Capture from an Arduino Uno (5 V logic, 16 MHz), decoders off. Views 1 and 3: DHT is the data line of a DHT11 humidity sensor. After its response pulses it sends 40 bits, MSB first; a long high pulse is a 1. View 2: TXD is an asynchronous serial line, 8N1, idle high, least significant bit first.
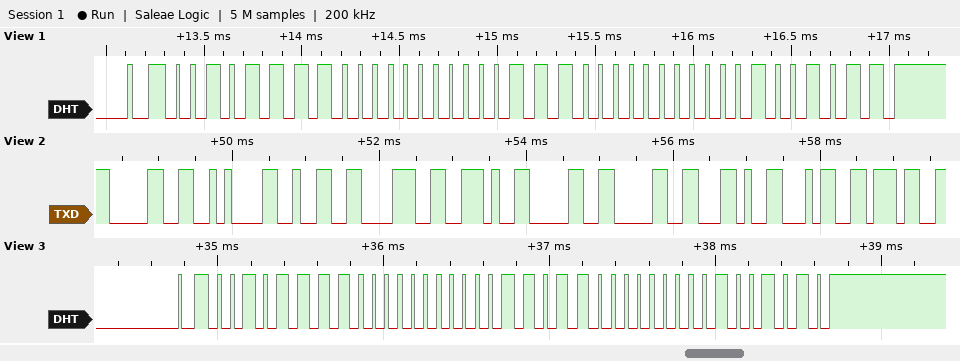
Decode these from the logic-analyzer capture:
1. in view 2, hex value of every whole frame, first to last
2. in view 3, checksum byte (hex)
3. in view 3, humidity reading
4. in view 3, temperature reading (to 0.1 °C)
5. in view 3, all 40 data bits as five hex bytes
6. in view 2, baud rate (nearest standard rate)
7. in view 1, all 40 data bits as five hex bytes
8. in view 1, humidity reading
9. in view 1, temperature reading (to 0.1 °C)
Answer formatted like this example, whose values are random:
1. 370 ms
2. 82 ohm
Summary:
1. 30 0A 32 38 2E 30 30 2C 34 37
2. 0x4A
3. 47 %
4. 27.0 °C
5. 2F 00 1B 00 4A
6. 9600 baud
7. 2F 00 1C 00 4B
8. 47 %
9. 28.0 °C
